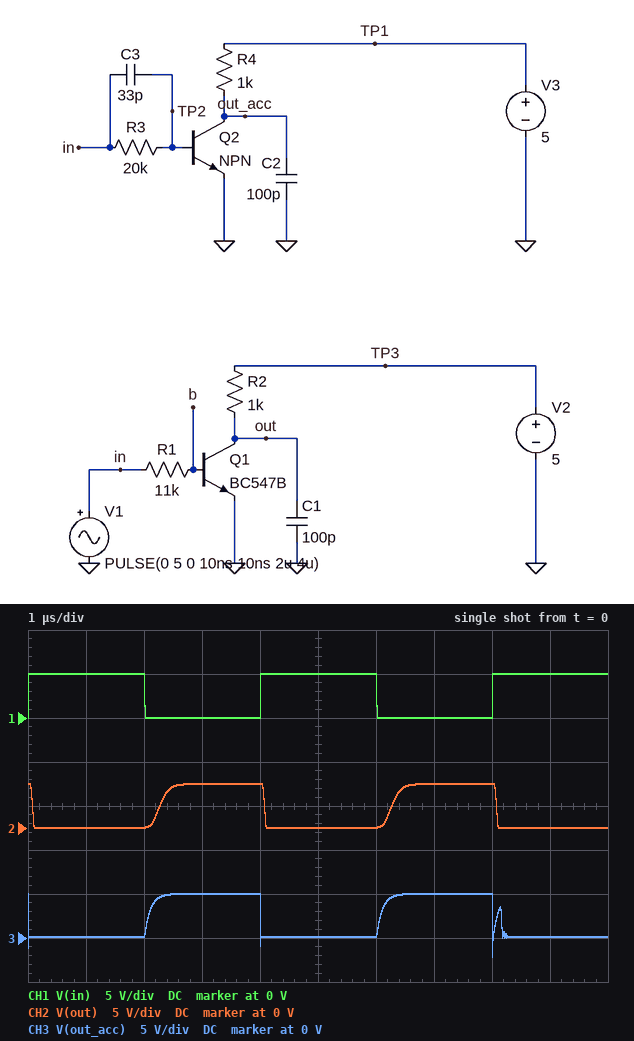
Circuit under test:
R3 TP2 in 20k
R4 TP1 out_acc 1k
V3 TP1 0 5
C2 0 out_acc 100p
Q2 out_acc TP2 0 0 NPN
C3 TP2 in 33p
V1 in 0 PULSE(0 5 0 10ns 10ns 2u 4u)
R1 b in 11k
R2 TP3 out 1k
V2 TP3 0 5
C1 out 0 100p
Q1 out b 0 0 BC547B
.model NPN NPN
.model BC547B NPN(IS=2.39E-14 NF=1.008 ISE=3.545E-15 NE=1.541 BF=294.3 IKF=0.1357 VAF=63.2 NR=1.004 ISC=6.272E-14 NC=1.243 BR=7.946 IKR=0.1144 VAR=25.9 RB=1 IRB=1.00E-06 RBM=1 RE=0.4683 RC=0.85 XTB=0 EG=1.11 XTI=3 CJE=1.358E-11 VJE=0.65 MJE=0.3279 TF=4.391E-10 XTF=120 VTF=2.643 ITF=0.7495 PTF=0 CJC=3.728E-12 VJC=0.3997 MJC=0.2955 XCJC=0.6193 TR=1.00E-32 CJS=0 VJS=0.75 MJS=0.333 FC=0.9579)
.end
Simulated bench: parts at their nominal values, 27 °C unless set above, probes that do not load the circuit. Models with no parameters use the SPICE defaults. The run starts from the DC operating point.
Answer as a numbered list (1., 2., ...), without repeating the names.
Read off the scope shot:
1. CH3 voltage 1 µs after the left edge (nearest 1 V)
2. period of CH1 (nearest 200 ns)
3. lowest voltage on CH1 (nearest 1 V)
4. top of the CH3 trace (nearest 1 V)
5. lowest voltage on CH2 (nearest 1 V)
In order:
1. 0 V
2. 4.0 µs
3. 0 V
4. 5 V
5. 0 V
